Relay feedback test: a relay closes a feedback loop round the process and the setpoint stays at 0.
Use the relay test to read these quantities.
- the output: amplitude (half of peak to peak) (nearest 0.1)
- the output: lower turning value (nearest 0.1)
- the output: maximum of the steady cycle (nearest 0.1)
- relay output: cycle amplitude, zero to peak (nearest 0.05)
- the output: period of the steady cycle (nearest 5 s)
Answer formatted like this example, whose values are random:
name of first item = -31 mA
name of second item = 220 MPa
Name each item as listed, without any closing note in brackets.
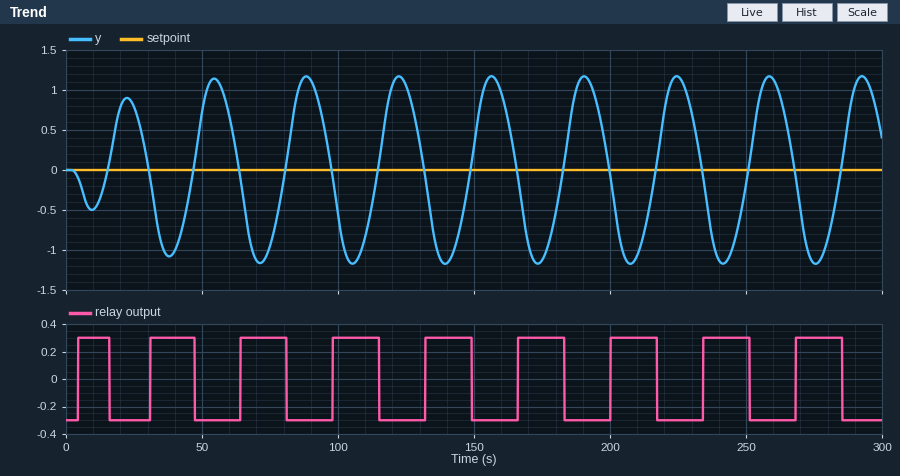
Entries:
the output: amplitude (half of peak to peak) = 1.2
the output: lower turning value = -1.2
the output: maximum of the steady cycle = 1.2
relay output: cycle amplitude, zero to peak = 0.30
the output: period of the steady cycle = 35 s
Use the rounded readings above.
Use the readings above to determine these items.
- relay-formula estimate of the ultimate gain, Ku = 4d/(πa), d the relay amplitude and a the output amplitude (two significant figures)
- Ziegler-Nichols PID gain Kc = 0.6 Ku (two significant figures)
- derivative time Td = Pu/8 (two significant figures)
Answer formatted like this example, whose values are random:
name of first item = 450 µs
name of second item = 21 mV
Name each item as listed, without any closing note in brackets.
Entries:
relay-formula estimate of the ultimate gain, Ku = 4d/(πa), d the relay amplitude and a the output amplitude = 0.32
Ziegler-Nichols PID gain Kc = 0.6 Ku = 0.19
derivative time Td = Pu/8 = 4.4 s
